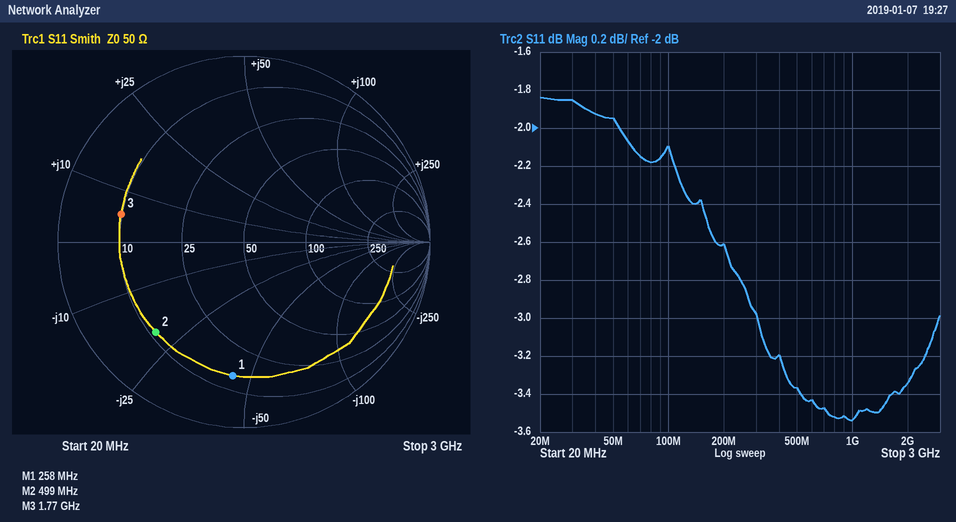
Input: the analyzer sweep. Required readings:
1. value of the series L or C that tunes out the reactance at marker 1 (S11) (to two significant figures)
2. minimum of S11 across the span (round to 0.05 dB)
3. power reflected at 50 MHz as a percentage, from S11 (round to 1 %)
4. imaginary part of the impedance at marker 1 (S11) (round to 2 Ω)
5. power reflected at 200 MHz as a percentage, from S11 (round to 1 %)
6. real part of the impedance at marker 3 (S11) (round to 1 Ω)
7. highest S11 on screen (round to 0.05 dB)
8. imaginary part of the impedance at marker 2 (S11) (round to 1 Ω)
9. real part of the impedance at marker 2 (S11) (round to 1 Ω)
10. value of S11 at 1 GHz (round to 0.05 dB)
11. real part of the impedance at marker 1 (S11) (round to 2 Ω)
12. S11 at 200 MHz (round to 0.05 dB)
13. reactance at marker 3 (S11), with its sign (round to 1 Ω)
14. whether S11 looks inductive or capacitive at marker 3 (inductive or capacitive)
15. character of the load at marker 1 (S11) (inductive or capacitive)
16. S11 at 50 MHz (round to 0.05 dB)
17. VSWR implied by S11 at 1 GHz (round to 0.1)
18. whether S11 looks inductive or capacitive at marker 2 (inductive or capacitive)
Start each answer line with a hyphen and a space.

- 27 nH
- -3.55 dB
- 64 %
- -44 Ω
- 55 %
- 10 Ω
- -1.85 dB
- -20 Ω
- 11 Ω
- -3.55 dB
- 14 Ω
- -2.60 dB
- +5 Ω
- inductive
- capacitive
- -1.95 dB
- 5.0
- capacitive
